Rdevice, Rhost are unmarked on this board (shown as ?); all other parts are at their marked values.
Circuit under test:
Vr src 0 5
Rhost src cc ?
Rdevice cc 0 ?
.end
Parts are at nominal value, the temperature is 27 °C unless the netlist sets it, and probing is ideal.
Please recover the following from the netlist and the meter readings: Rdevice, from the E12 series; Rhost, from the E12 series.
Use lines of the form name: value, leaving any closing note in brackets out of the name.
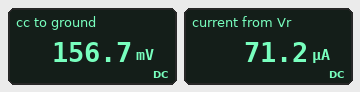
Rdevice, from the E12 series: 2.2 kΩ
Rhost, from the E12 series: 68 kΩ
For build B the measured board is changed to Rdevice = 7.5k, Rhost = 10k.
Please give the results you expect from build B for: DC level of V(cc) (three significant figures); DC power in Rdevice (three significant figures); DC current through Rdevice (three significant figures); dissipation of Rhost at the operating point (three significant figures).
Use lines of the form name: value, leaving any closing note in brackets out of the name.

DC level of V(cc): 2.14 V
DC power in Rdevice: 612 µW
DC current through Rdevice: 286 µA
dissipation of Rhost at the operating point: 816 µW
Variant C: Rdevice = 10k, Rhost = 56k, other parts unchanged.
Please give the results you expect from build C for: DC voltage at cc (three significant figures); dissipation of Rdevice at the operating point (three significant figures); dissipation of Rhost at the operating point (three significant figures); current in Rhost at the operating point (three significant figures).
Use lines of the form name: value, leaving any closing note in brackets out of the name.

DC voltage at cc: 758 mV
dissipation of Rdevice at the operating point: 57.4 µW
dissipation of Rhost at the operating point: 321 µW
current in Rhost at the operating point: 75.8 µA
